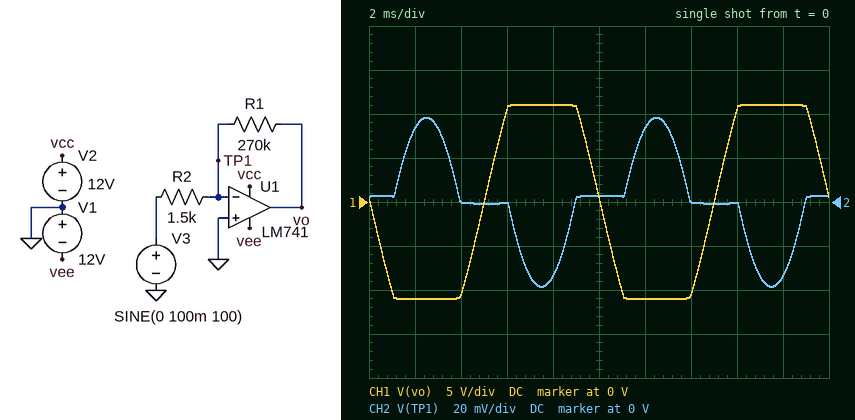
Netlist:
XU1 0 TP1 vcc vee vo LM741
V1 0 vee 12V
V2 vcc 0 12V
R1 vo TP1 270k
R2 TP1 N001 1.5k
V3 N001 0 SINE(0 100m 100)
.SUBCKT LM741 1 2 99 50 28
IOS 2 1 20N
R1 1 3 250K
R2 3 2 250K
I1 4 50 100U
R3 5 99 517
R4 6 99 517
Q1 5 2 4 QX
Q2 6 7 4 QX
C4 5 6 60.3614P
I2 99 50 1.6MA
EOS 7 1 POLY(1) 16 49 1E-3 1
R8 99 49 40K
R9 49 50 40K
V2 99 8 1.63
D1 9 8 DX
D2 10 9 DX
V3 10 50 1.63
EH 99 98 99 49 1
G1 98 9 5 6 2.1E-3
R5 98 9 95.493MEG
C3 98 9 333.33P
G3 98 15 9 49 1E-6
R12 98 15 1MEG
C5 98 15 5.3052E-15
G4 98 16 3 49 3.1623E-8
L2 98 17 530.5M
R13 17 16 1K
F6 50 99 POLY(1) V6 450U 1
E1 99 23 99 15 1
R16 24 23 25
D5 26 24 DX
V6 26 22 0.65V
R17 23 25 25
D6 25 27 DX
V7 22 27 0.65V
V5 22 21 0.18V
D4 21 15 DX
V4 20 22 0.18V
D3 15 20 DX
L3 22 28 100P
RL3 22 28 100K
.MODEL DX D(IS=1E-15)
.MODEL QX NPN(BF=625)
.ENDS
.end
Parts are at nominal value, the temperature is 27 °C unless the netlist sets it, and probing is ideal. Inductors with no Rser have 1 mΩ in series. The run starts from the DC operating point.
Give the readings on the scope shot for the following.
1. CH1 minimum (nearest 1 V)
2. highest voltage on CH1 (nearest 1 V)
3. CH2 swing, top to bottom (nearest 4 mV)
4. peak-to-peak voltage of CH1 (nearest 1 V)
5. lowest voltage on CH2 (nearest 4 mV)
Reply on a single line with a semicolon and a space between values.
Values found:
-11 V; 11 V; 76 mV; 22 V; -40 mV
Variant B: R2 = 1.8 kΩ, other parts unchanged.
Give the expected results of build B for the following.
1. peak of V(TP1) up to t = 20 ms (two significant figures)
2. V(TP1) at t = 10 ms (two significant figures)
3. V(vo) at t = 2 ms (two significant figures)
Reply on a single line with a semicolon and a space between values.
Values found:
26 mV; 2.5 mV; -11 V
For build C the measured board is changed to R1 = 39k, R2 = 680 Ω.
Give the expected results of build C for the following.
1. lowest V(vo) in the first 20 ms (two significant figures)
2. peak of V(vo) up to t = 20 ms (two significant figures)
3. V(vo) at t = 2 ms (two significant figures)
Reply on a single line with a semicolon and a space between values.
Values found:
-5.7 V; 5.8 V; -5.4 V
